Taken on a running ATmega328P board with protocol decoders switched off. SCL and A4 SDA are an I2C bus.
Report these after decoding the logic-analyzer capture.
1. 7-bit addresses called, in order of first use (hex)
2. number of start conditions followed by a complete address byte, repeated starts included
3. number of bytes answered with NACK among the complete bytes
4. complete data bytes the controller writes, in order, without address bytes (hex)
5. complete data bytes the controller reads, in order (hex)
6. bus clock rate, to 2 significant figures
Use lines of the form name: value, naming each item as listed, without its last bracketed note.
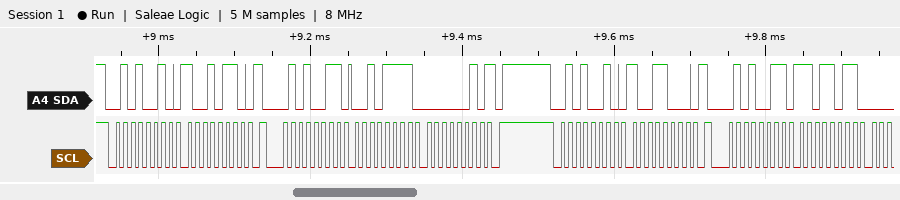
7-bit addresses called, in order of first use: 0x29
number of start conditions followed by a complete address byte, repeated starts included: 4
number of bytes answered with NACK among the complete bytes: 1
complete data bytes the controller writes, in order, without address bytes: 96 98
complete data bytes the controller reads, in order: 2F 02 DB
bus clock rate, to 2 significant figures: 100 kHz
